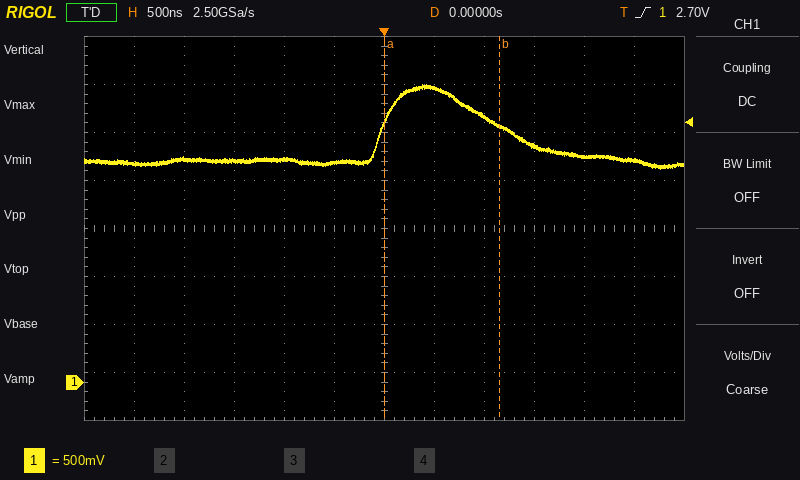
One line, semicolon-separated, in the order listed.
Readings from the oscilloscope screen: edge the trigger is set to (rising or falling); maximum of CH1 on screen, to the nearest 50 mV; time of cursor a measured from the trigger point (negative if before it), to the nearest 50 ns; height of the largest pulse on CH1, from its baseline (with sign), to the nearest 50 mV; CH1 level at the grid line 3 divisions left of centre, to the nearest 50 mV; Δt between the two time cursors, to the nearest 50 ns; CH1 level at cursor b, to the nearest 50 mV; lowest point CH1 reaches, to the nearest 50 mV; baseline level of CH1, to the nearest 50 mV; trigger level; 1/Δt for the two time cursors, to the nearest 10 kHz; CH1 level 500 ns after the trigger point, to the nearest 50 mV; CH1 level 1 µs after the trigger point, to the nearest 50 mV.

rising; 3.10 V; 0 ns; +800 mV; 2.30 V; 1.15 µs; 2.65 V; 2.20 V; 2.30 V; 2.70 V; 870 kHz; 3.05 V; 2.75 V
